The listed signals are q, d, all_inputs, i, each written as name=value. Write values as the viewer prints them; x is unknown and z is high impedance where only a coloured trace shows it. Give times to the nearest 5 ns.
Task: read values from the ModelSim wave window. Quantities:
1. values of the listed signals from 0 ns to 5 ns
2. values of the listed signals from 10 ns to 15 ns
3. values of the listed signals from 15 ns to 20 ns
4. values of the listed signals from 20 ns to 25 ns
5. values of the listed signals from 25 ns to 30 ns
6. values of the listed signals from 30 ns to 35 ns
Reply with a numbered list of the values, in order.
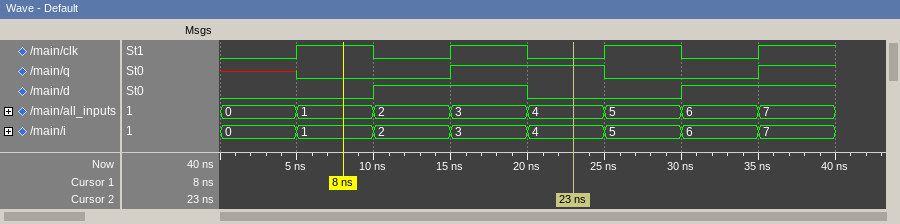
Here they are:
1. q=x, d=0, all_inputs=0, i=0
2. q=0, d=1, all_inputs=2, i=2
3. q=1, d=1, all_inputs=3, i=3
4. q=1, d=0, all_inputs=4, i=4
5. q=0, d=0, all_inputs=5, i=5
6. q=0, d=1, all_inputs=6, i=6
